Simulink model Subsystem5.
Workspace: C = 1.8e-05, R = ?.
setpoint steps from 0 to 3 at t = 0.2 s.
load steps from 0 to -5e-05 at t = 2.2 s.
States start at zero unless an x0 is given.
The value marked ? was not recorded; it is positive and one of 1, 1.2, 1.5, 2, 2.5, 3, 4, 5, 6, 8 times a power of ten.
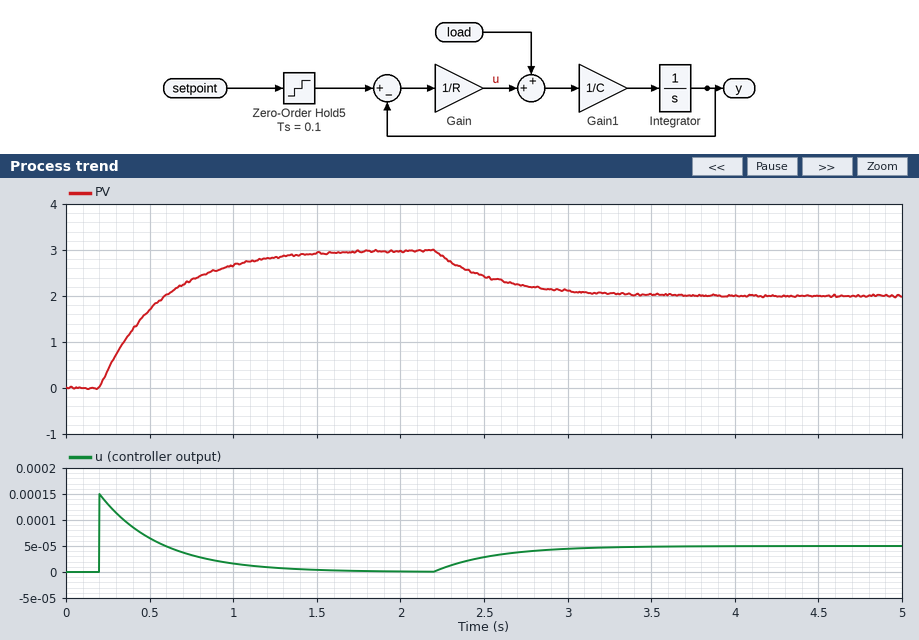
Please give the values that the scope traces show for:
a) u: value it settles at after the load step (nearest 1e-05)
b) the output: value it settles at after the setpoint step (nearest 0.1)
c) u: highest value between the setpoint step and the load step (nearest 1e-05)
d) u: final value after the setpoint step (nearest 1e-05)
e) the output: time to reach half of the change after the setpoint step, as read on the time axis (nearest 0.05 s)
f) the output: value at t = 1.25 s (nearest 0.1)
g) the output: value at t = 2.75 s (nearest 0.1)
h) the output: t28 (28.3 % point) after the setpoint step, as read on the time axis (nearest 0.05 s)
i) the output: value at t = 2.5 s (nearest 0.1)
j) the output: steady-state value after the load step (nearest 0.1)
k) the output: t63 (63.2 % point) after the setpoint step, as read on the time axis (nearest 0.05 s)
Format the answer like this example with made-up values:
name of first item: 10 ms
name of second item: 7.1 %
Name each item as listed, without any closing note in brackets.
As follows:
u: value it settles at after the load step: 0.00005
the output: value it settles at after the setpoint step: 3.0
u: highest value between the setpoint step and the load step: 0.00015
u: final value after the setpoint step: 0.00000
the output: time to reach half of the change after the setpoint step, as read on the time axis: 0.45 s
the output: value at t = 1.25 s: 2.8
the output: value at t = 2.75 s: 2.2
the output: t28 (28.3 % point) after the setpoint step, as read on the time axis: 0.30 s
the output: value at t = 2.5 s: 2.4
the output: steady-state value after the load step: 2.0
the output: t63 (63.2 % point) after the setpoint step, as read on the time axis: 0.55 s
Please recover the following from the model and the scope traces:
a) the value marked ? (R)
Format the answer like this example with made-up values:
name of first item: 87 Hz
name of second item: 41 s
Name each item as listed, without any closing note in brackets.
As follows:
the value marked ?: 20000
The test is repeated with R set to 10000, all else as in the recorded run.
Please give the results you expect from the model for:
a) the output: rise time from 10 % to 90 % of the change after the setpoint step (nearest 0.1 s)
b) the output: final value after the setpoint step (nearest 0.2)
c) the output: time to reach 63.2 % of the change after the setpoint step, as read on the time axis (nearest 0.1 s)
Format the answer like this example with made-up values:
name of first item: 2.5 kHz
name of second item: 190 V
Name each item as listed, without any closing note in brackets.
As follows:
the output: rise time from 10 % to 90 % of the change after the setpoint step: 0.4 s
the output: final value after the setpoint step: 3.0
the output: time to reach 63.2 % of the change after the setpoint step, as read on the time axis: 0.4 s
